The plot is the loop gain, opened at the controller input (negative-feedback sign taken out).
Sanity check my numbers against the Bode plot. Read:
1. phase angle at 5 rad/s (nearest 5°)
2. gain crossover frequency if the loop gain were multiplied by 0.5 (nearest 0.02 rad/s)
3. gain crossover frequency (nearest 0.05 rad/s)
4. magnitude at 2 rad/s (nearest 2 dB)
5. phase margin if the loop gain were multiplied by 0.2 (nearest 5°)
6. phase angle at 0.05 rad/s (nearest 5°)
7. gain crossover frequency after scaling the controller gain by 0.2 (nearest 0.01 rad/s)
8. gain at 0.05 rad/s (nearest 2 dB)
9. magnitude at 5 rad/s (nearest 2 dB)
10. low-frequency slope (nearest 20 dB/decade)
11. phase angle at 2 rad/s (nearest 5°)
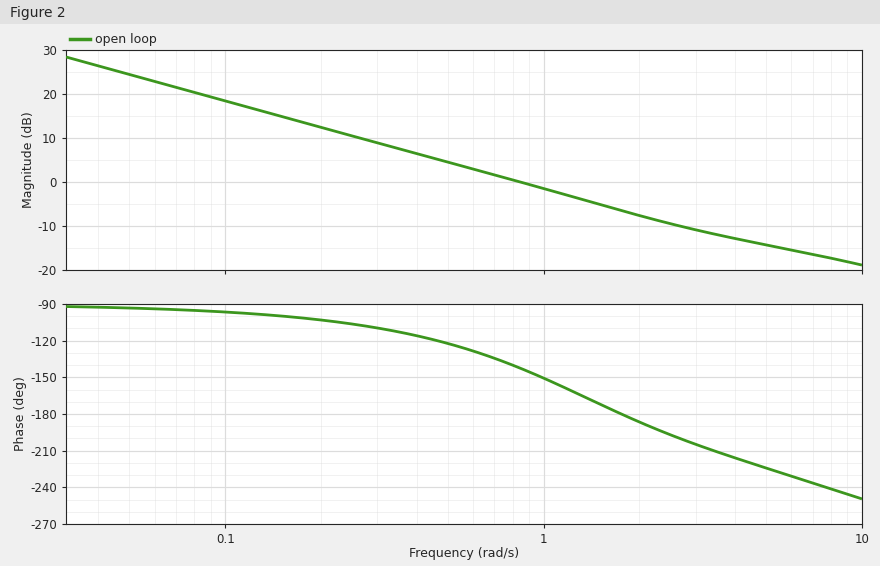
-225°
0.42 rad/s
0.85 rad/s
-8 dB
80°
-95°
0.17 rad/s
24 dB
-14 dB
-20 dB/decade
-185°
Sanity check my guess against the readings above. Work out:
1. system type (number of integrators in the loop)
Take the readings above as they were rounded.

1
